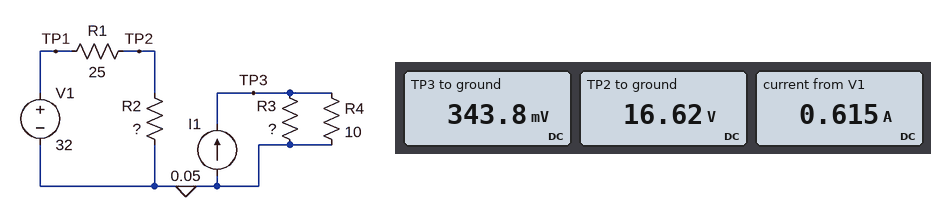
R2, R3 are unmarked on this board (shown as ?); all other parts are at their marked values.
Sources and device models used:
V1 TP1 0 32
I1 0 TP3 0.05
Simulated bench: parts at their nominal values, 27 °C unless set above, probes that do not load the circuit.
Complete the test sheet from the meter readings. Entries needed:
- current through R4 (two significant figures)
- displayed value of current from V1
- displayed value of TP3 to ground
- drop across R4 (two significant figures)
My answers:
34 mA
0.615 A
343.8 mV
340 mV
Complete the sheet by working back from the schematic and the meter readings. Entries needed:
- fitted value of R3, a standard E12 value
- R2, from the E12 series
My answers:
22 Ω
27 Ω
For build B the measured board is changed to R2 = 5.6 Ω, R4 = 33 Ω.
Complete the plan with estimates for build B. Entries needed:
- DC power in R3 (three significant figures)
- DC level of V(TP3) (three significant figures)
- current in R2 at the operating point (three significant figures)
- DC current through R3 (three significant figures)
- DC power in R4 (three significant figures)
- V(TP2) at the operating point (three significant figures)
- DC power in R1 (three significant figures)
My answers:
19.8 mW
660 mV
1.05 A
30.0 mA
13.2 mW
5.86 V
27.3 W
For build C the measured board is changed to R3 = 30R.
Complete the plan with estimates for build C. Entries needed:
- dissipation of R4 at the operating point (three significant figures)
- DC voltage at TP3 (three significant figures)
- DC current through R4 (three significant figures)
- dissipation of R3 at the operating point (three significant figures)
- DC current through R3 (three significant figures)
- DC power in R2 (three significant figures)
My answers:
14.1 mW
375 mV
37.5 mA
4.69 mW
12.5 mA
10.2 W
